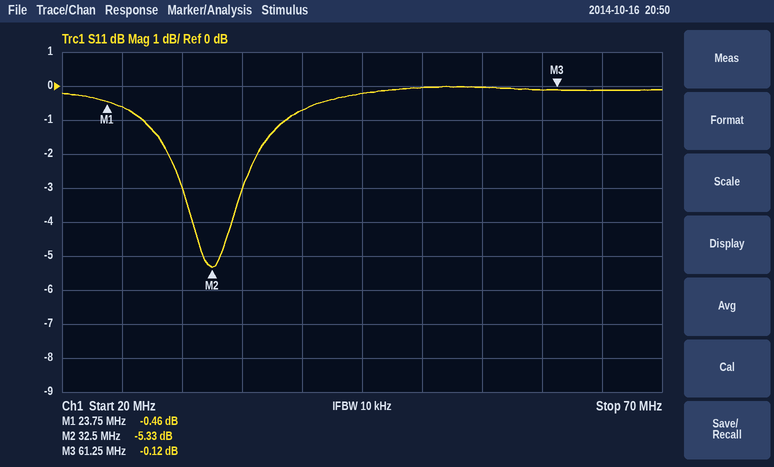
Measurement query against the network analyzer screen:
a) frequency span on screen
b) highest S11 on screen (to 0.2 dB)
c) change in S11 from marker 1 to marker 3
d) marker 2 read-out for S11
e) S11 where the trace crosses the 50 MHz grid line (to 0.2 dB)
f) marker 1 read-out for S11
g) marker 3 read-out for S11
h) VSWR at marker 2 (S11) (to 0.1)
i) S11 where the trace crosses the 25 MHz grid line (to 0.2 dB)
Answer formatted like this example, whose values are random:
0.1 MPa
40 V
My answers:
50 MHz
0.0 dB
0.34 dB
-5.33 dB
0.0 dB
-0.46 dB
-0.12 dB
3.4
-0.6 dB
